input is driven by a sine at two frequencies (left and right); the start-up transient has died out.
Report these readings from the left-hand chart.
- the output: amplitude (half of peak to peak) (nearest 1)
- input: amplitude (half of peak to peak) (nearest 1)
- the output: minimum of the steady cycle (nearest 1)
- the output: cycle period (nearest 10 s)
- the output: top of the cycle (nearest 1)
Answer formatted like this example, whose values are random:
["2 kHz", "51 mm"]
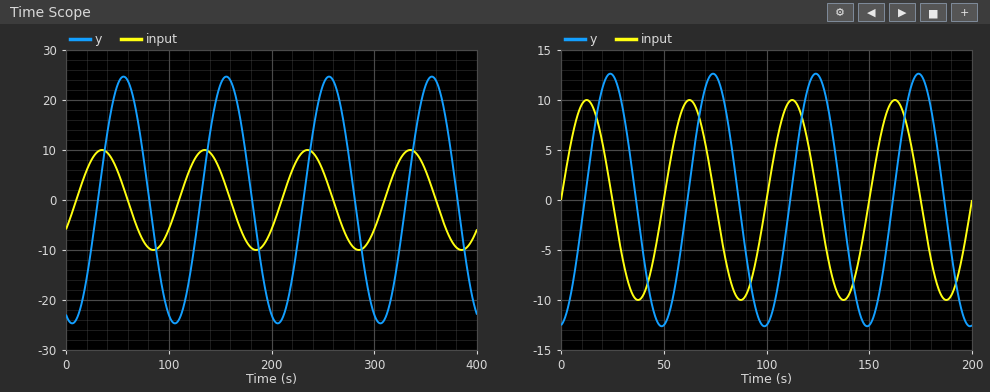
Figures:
["25", "10", "-25", "100 s", "25"]
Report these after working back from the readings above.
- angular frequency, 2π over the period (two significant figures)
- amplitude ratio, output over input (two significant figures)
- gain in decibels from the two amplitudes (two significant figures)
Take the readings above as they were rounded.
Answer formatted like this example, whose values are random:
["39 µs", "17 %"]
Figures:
["0.063 rad/s", "2.5", "8.0 dB"]
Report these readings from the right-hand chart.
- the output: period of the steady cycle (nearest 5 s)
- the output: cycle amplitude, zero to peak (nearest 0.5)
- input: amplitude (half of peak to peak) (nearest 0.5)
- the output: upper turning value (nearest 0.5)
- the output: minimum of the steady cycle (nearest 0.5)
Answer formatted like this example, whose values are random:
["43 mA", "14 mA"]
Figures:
["50 s", "12.5", "10.0", "12.5", "-12.5"]
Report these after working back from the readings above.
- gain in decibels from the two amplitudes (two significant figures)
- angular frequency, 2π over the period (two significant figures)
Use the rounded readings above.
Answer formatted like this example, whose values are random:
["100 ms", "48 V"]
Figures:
["1.9 dB", "0.13 rad/s"]
